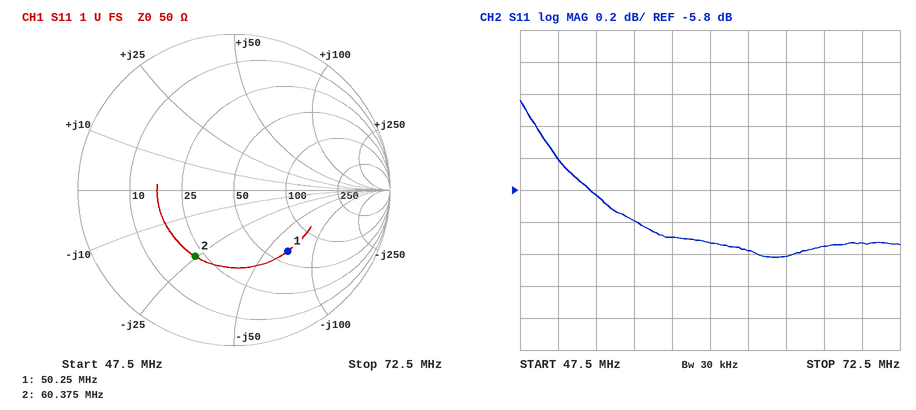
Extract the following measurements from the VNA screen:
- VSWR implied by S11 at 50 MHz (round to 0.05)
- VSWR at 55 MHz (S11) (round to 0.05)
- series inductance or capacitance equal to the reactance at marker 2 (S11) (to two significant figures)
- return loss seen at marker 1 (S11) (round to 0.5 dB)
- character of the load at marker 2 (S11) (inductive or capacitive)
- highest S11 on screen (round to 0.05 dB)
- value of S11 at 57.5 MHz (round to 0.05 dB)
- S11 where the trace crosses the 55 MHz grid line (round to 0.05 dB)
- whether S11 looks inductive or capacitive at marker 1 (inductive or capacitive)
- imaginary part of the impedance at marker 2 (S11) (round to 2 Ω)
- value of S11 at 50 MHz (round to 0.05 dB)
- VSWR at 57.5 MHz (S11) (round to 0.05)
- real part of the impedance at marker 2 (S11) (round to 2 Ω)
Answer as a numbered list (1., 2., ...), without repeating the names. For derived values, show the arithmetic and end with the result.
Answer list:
1. |Γ| = 10^(-5.6/20) = 0.5248; VSWR = (1 + 0.5248)/(1 − 0.5248) ≈ 3.21, so 3.20 to the nearest 0.05
2. |Γ| = 10^(-6/20) = 0.5012; VSWR = (1 + 0.5012)/(1 − 0.5012) ≈ 3.01, so 3.00 to the nearest 0.05
3. C = 1/(2π × 60.375 MHz × 24 Ω) ≈ 110 pF
4. 5.5 dB
5. capacitive
6. -5.25 dB
7. -6.10 dB
8. -6.00 dB
9. capacitive
10. -24 Ω
11. -5.60 dB
12. |Γ| = 10^(-6.1/20) = 0.4955; VSWR = (1 + 0.4955)/(1 − 0.4955) ≈ 2.96, so 2.95 to the nearest 0.05
13. 22 Ω
